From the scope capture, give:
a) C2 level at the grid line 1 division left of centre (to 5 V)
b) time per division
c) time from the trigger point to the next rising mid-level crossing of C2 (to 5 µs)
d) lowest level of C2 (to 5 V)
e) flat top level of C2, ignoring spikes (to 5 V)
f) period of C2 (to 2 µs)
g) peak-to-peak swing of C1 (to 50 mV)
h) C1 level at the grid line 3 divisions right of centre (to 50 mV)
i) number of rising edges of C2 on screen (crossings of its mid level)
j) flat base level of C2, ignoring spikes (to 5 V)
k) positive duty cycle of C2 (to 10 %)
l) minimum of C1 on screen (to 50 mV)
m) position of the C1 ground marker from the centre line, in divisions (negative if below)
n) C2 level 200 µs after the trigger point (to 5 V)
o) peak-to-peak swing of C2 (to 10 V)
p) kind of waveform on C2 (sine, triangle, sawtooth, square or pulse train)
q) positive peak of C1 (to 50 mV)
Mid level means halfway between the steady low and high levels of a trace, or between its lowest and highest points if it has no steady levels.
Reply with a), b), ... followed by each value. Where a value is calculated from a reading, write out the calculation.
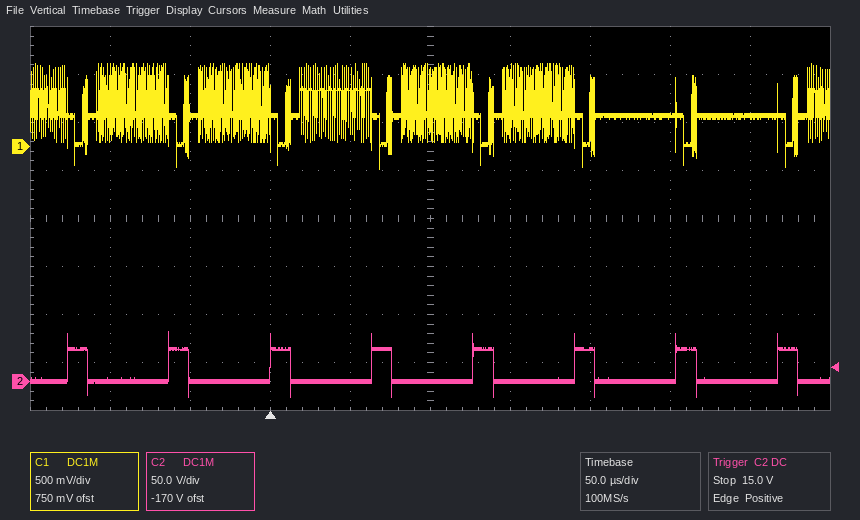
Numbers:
a) 0 V
b) 50 µs
c) 65 µs
d) -15 V
e) 35 V
f) 64 µs
g) 850 mV − (-250 mV) = 1.10 V
h) 300 mV
i) 8
j) 0 V
k) 20 %
l) -250 mV
m) +1.5 div
n) 35 V
o) 70 V
p) pulse train
q) 850 mV
